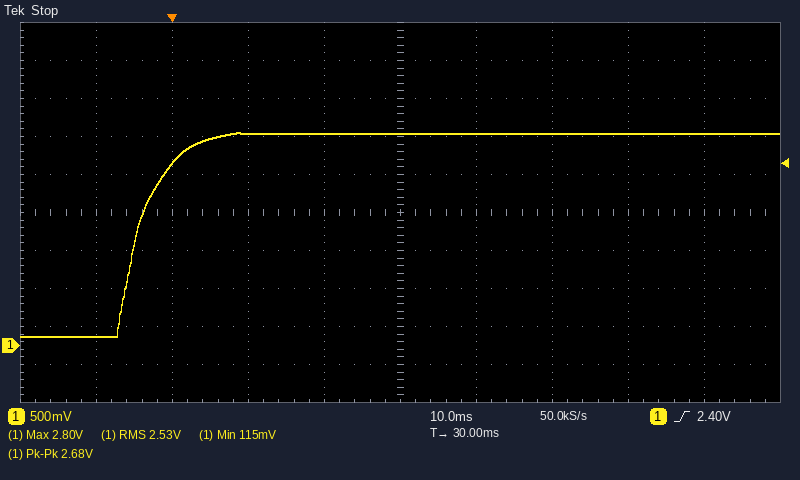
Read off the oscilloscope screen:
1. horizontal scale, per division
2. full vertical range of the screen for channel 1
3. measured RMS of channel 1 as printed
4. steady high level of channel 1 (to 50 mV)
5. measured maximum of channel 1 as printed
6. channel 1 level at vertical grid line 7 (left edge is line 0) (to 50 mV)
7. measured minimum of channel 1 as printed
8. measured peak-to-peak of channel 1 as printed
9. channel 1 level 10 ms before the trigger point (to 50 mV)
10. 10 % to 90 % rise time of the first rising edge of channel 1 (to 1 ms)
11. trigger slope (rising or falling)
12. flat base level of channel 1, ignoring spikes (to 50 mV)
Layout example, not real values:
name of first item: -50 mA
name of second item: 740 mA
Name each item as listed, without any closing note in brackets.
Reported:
horizontal scale, per division: 10 ms
full vertical range of the screen for channel 1: 5 V
measured RMS of channel 1 as printed: 2.53 V
steady high level of channel 1: 2.80 V
measured maximum of channel 1 as printed: 2.80 V
channel 1 level at vertical grid line 7 (left edge is line 0): 2.80 V
measured minimum of channel 1 as printed: 115 mV
measured peak-to-peak of channel 1 as printed: 2.68 V
channel 1 level 10 ms before the trigger point: 100 mV
10 % to 90 % rise time of the first rising edge of channel 1: 8 ms
trigger slope: rising
flat base level of channel 1, ignoring spikes: 100 mV
